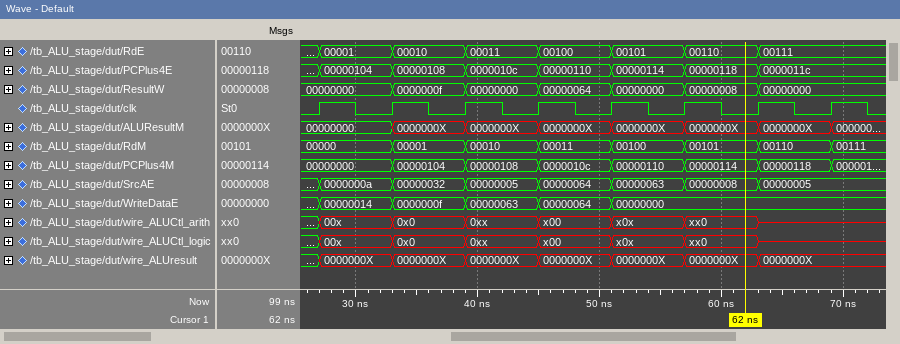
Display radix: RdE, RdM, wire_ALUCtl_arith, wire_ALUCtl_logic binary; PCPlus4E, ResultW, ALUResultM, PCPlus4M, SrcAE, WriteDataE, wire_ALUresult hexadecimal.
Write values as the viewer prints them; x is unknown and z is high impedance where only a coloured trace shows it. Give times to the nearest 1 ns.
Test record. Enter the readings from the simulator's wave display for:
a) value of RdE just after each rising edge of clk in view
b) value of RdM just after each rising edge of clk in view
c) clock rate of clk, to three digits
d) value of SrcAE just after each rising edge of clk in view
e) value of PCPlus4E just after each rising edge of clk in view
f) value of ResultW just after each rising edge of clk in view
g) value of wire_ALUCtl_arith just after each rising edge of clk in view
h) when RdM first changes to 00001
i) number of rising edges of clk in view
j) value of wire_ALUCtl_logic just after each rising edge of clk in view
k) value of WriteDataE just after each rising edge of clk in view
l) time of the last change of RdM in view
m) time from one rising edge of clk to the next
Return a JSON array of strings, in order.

["00001, 00010, 00011, 00100, 00101, 00110, 00111, 00111", "00000, 00001, 00010, 00011, 00100, 00101, 00110, 00111", "167 MHz", "0000000a, 00000032, 00000005, 00000064, 00000063, 00000008, 00000005, 00000005", "00000104, 00000108, 0000010c, 00000110, 00000114, 00000118, 0000011c, 0000011c", "00000000, 0000000f, 00000000, 00000064, 00000000, 00000008, 00000000, 00000000", "00x, 0x0, 0xx, x00, x0x, xx0, x, x", "33 ns", "8", "00x, 0x0, 0xx, x00, x0x, xx0, x, x", "00000014, 0000000f, 00000063, 00000064, 00000000, 00000000, 00000000, 00000000", "69 ns", "6 ns"]
